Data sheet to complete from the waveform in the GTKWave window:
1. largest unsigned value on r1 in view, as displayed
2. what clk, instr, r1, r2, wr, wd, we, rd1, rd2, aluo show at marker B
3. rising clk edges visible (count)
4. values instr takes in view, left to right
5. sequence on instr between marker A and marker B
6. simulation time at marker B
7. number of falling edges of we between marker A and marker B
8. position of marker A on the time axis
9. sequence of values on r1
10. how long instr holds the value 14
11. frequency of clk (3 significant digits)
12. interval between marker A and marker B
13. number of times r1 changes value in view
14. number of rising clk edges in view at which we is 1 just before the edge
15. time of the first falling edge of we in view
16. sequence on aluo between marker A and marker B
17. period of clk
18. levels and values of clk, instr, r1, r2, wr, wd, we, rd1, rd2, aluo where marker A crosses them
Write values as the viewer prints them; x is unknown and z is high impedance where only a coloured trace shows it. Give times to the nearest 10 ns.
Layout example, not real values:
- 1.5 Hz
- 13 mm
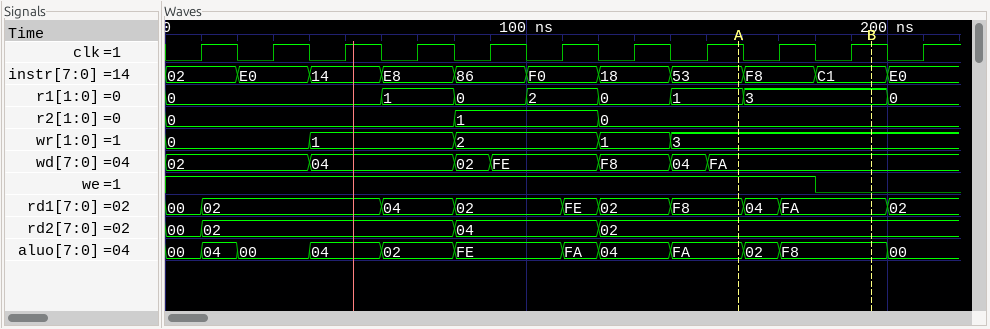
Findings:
- 3
- clk=1, instr=C1, r1=3, r2=0, wr=3, wd=FA, we=0, rd1=FA, rd2=02, aluo=F8
- 11
- 02, E0, 14, E8, 86, F0, 18, 53, F8, C1, E0
- 53, F8, C1
- 200 ns
- 1
- 160 ns
- 0, 1, 0, 2, 0, 1, 3, 0
- 20 ns
- 50.0 MHz
- 40 ns
- 7
- 9
- 180 ns
- FA, 02, F8
- 20 ns
- clk=1, instr=53, r1=1, r2=0, wr=3, wd=FA, we=1, rd1=F8, rd2=02, aluo=FA
